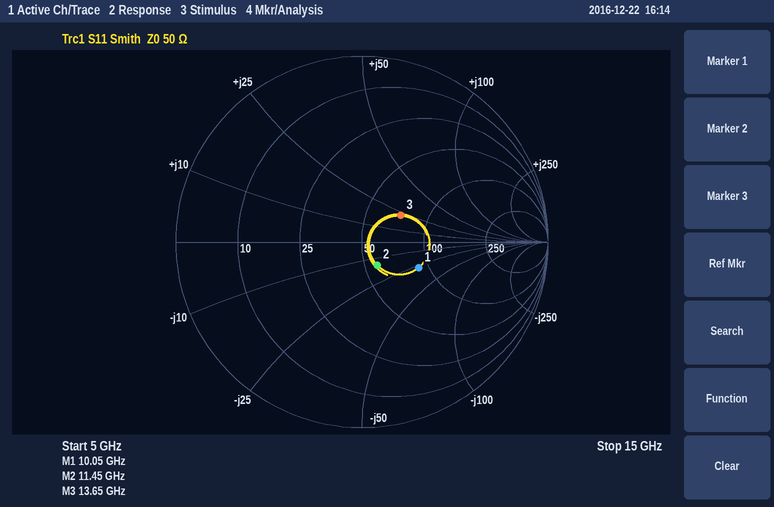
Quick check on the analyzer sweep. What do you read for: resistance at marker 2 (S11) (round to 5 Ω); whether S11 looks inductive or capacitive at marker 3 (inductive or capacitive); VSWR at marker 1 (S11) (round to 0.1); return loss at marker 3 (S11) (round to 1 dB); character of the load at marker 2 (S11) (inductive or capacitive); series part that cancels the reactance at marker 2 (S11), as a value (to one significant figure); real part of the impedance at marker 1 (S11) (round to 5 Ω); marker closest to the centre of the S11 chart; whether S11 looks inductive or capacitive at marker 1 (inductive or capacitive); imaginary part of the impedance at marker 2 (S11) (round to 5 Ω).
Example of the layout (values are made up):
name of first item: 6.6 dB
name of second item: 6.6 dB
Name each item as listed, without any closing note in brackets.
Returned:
resistance at marker 2 (S11): 55 Ω
whether S11 looks inductive or capacitive at marker 3: inductive
VSWR at marker 1 (S11): 2.0
return loss at marker 3 (S11): 12 dB
character of the load at marker 2 (S11): capacitive
series part that cancels the reactance at marker 2 (S11), as a value: 200 pH
real part of the impedance at marker 1 (S11): 90 Ω
marker closest to the centre of the S11 chart: marker 2
whether S11 looks inductive or capacitive at marker 1: capacitive
imaginary part of the impedance at marker 2 (S11): -15 Ω
